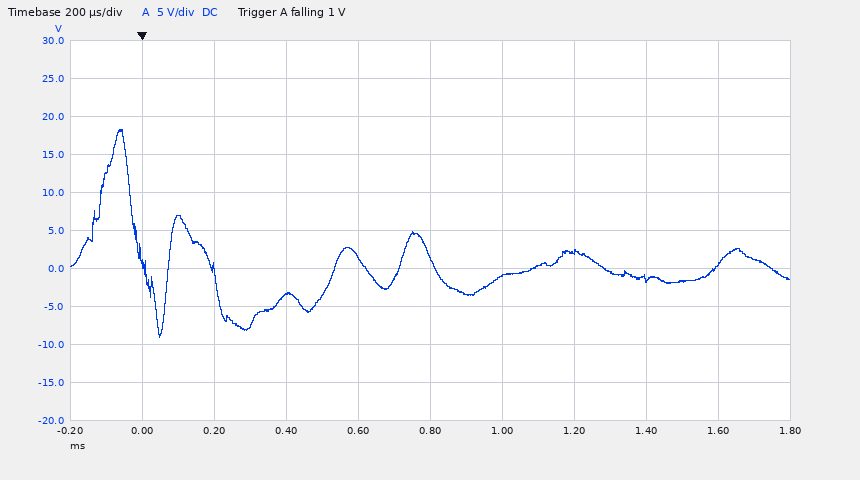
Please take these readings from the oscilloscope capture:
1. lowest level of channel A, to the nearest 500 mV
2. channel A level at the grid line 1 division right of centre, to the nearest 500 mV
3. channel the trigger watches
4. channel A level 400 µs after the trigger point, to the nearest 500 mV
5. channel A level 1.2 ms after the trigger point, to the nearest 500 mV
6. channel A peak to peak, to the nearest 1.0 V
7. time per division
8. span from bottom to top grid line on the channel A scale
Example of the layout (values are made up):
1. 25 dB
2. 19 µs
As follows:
1. -9.0 V
2. -1.0 V
3. channel A
4. -3.5 V
5. 2.0 V
6. 27.0 V
7. 200 µs
8. 50 V
